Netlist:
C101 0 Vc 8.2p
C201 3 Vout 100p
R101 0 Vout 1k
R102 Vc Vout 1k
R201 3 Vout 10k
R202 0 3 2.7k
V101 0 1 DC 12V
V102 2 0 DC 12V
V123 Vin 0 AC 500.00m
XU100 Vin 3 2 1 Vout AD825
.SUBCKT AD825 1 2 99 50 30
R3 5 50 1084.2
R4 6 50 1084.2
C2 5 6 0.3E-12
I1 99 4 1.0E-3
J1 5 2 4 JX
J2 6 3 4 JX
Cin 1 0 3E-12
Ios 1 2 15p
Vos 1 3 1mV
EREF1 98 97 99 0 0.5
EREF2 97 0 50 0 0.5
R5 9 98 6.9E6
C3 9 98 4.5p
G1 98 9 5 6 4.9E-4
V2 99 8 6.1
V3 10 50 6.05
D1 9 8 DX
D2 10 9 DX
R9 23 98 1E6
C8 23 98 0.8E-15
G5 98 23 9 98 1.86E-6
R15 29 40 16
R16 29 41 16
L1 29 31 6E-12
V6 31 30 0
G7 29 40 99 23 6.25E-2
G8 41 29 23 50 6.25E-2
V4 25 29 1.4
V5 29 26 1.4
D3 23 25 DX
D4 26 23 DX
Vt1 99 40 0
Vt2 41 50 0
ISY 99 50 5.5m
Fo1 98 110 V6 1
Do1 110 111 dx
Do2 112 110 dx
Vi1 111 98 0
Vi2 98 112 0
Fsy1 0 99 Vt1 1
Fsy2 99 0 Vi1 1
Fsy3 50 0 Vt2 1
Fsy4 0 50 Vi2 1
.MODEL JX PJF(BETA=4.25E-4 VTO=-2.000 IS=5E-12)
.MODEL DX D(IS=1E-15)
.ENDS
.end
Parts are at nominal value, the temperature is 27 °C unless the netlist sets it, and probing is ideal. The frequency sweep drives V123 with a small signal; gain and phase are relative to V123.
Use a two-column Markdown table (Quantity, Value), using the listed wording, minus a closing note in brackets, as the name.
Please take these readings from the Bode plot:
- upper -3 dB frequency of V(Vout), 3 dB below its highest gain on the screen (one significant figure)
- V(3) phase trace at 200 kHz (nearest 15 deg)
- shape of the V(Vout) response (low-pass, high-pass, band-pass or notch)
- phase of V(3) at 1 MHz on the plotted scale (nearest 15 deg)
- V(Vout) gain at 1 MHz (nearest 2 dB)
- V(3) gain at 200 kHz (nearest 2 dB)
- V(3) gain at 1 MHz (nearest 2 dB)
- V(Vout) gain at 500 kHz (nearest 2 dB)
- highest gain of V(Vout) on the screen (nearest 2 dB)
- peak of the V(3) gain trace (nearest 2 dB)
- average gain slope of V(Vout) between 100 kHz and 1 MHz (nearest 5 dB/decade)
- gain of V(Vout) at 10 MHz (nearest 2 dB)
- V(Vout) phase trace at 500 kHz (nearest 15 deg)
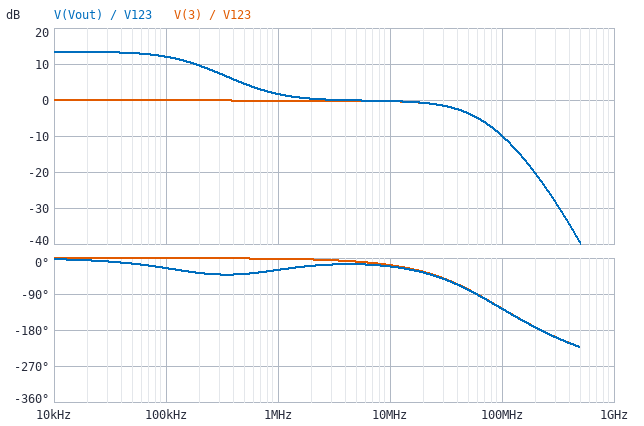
| Quantity | Value |
|---|---|
| upper -3 dB frequency of V(Vout), 3 dB below its highest gain on the screen | 200 kHz |
| V(3) phase trace at 200 kHz | 0 deg |
| shape of the V(Vout) response | low-pass |
| phase of V(3) at 1 MHz on the plotted scale | 0 deg |
| V(Vout) gain at 1 MHz | 2 dB |
| V(3) gain at 200 kHz | 0 dB |
| V(3) gain at 1 MHz | 0 dB |
| V(Vout) gain at 500 kHz | 4 dB |
| highest gain of V(Vout) on the screen | 14 dB |
| peak of the V(3) gain trace | 0 dB |
| average gain slope of V(Vout) between 100 kHz and 1 MHz | -10 dB/decade |
| gain of V(Vout) at 10 MHz | 0 dB |
| V(Vout) phase trace at 500 kHz | -45 deg |
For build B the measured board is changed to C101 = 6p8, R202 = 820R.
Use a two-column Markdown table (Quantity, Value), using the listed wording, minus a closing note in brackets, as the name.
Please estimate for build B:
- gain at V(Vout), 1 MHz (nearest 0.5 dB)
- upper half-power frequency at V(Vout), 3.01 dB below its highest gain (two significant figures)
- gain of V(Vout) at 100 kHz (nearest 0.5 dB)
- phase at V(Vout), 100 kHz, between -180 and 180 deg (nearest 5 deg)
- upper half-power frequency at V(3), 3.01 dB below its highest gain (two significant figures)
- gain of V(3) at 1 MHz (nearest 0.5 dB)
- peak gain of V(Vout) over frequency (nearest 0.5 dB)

| Quantity | Value |
|---|---|
| gain at V(Vout), 1 MHz | 6.5 dB |
| upper half-power frequency at V(Vout), 3.01 dB below its highest gain | 150 kHz |
| gain of V(Vout) at 100 kHz | 21.0 dB |
| phase at V(Vout), 100 kHz, between -180 and 180 deg | -30 deg |
| upper half-power frequency at V(3), 3.01 dB below its highest gain | 42 MHz |
| gain of V(3) at 1 MHz | -0.5 dB |
| peak gain of V(Vout) over frequency | 22.5 dB |
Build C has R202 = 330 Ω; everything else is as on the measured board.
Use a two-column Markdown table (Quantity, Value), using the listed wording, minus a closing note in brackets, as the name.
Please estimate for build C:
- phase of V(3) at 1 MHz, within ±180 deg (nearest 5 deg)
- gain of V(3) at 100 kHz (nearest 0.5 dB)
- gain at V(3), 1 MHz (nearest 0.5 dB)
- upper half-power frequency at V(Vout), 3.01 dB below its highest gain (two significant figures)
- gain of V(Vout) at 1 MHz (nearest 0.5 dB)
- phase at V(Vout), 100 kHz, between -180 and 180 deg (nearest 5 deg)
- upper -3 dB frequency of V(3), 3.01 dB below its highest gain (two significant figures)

| Quantity | Value |
|---|---|
| phase of V(3) at 1 MHz, within ±180 deg | -5 deg |
| gain of V(3) at 100 kHz | -0.5 dB |
| gain at V(3), 1 MHz | -1.0 dB |
| upper half-power frequency at V(Vout), 3.01 dB below its highest gain | 140 kHz |
| gain of V(Vout) at 1 MHz | 13.0 dB |
| phase at V(Vout), 100 kHz, between -180 and 180 deg | -35 deg |
| upper -3 dB frequency of V(3), 3.01 dB below its highest gain | 37 MHz |
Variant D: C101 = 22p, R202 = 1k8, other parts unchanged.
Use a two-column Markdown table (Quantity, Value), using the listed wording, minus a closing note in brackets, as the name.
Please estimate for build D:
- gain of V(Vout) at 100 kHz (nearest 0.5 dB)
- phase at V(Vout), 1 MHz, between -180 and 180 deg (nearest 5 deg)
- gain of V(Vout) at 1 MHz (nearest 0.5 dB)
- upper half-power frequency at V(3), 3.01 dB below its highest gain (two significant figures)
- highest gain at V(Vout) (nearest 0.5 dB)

| Quantity | Value |
|---|---|
| gain of V(Vout) at 100 kHz | 15.0 dB |
| phase at V(Vout), 1 MHz, between -180 and 180 deg | -40 deg |
| gain of V(Vout) at 1 MHz | 3.0 dB |
| upper half-power frequency at V(3), 3.01 dB below its highest gain | 43 MHz |
| highest gain at V(Vout) | 16.5 dB |
